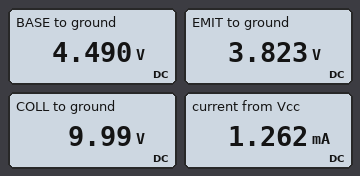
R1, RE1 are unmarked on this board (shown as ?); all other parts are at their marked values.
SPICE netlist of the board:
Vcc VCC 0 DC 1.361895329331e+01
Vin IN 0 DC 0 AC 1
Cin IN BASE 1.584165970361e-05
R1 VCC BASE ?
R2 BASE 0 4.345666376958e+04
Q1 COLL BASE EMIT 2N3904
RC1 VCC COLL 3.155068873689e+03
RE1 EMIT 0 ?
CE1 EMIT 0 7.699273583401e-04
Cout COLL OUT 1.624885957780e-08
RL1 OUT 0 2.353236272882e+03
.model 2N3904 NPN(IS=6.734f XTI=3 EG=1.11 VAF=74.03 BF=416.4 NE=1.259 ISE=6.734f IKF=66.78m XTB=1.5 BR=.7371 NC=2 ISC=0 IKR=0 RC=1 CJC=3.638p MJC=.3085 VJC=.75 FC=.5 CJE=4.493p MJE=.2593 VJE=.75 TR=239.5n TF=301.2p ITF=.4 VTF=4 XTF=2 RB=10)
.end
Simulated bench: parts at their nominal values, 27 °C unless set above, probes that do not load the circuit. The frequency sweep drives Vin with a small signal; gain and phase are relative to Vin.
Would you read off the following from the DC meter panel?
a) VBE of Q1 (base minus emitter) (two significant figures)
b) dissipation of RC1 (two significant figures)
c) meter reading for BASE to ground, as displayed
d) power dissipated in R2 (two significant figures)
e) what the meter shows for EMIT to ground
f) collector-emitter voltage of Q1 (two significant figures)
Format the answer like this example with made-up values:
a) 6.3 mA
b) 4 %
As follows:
a) 670 mV
b) 4.2 mW
c) 4.490 V
d) 460 µW
e) 3.823 V
f) 6.2 V
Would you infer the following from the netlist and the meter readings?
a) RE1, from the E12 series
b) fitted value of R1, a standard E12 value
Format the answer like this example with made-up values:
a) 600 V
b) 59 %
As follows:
a) 3.3 kΩ
b) 82 kΩ
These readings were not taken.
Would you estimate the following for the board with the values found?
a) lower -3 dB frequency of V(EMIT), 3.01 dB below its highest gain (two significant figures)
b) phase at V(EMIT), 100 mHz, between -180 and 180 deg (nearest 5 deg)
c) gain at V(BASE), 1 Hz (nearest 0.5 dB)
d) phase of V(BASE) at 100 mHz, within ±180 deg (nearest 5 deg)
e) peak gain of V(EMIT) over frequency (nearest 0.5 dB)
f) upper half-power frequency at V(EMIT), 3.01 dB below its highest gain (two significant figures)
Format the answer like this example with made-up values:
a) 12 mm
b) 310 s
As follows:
a) 270 mHz
b) 70 deg
c) -2.5 dB
d) 70 deg
e) -2.5 dB
f) 12 Hz
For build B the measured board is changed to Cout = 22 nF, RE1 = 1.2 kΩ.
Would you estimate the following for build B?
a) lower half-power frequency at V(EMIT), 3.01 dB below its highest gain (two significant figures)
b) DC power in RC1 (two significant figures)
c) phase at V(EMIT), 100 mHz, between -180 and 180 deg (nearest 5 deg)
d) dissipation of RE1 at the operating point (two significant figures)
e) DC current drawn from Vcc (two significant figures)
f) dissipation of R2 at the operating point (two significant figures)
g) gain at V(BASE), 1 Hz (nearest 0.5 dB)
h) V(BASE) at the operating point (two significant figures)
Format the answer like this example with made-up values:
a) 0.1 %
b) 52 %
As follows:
a) 300 mHz
b) 26 mW
c) 70 deg
d) 10 mW
e) 3.0 mA
f) 400 µW
g) -3.0 dB
h) 4.2 V
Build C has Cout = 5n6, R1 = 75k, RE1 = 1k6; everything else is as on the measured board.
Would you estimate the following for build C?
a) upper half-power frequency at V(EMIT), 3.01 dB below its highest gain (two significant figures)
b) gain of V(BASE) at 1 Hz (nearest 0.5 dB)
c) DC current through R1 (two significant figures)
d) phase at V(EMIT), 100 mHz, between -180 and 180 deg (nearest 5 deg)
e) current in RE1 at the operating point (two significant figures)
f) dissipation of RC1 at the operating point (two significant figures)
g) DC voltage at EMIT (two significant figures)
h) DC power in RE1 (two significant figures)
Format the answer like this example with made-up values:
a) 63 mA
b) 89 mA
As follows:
a) 23 Hz
b) -3.0 dB
c) 120 µA
d) 70 deg
e) 2.4 mA
f) 18 mW
g) 3.9 V
h) 9.3 mW
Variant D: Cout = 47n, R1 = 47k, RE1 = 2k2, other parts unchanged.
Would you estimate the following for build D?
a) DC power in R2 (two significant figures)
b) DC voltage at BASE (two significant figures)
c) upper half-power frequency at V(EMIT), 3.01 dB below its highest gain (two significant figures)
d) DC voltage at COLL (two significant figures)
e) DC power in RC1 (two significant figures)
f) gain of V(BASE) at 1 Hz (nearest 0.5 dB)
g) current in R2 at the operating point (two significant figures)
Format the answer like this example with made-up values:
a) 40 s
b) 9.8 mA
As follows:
a) 870 µW
b) 6.2 V
c) 24 Hz
d) 5.8 V
e) 19 mW
f) -3.0 dB
g) 140 µA
